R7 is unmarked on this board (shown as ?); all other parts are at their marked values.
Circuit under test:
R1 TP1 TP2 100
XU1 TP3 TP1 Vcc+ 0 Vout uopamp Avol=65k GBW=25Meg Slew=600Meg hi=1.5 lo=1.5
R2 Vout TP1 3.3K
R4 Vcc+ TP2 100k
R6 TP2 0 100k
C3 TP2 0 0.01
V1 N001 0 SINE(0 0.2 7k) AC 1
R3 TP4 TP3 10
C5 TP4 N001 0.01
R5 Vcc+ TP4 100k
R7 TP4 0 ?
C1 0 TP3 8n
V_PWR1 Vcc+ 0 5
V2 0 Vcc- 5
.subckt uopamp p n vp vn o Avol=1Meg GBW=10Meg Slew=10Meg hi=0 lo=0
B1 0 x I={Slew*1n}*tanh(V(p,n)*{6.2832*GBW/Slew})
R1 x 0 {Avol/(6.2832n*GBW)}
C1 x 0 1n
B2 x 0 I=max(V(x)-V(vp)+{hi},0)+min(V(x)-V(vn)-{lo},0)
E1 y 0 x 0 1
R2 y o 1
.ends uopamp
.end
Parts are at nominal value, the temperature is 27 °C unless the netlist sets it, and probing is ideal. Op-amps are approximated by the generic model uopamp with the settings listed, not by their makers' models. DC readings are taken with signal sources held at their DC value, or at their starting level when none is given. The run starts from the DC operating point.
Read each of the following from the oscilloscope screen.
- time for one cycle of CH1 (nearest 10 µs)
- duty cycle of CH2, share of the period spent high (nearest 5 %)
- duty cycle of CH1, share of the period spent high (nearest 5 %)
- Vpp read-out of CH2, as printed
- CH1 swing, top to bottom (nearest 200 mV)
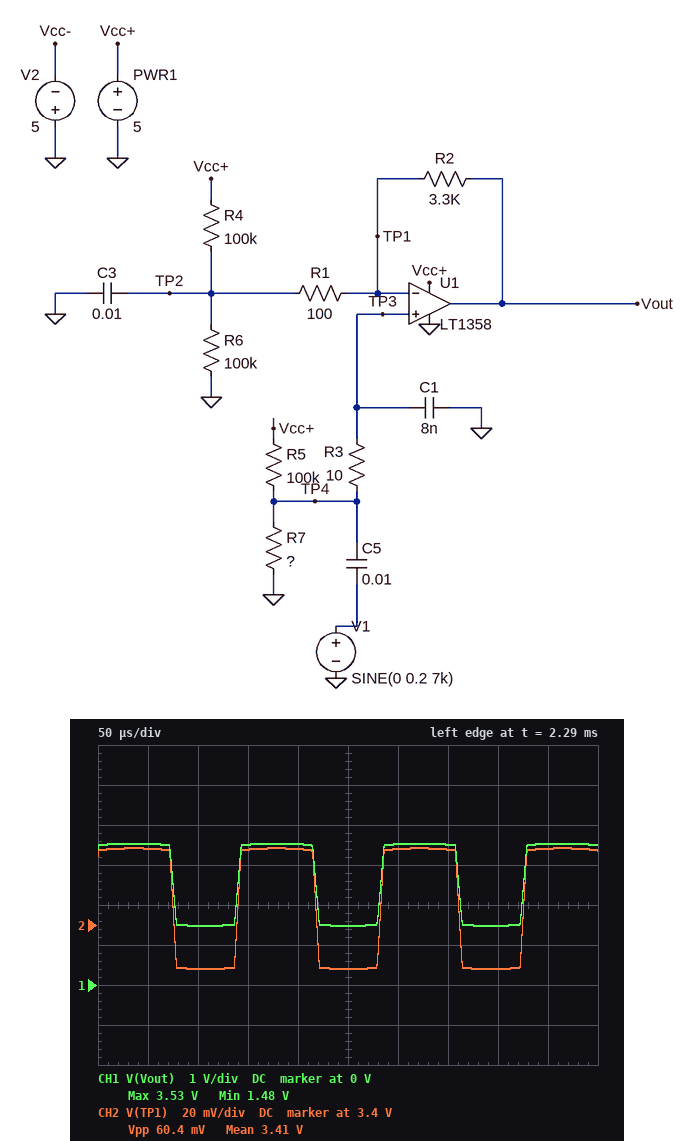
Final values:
140 µs
55 %
55 %
60.4 mV
2.0 V
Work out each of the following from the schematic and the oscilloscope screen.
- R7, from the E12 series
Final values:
220 kΩ
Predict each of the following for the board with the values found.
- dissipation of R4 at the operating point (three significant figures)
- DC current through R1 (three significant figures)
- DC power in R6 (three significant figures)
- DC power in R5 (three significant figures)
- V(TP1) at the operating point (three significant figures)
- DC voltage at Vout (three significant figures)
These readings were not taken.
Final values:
24.5 µW
18.7 µA
118 µW
24.4 µW
3.44 V
3.50 V
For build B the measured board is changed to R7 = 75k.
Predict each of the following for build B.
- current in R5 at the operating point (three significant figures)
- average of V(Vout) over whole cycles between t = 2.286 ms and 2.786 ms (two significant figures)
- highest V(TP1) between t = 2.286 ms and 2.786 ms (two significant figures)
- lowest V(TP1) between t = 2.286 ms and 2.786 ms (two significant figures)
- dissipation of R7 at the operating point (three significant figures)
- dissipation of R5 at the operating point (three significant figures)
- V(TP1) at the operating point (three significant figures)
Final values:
28.6 µA
2.5 V
2.2 V
2.1 V
61.2 µW
81.6 µW
2.14 V
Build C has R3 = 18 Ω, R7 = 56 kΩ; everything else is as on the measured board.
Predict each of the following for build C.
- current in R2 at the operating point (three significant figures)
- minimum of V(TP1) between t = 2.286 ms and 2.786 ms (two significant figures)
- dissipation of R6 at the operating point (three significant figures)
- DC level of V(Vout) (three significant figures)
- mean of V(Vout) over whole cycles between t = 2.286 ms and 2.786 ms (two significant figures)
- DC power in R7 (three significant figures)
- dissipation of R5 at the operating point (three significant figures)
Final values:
14.1 µA
1.8 V
32.3 µW
1.75 V
2.4 V
57.5 µW
103 µW
